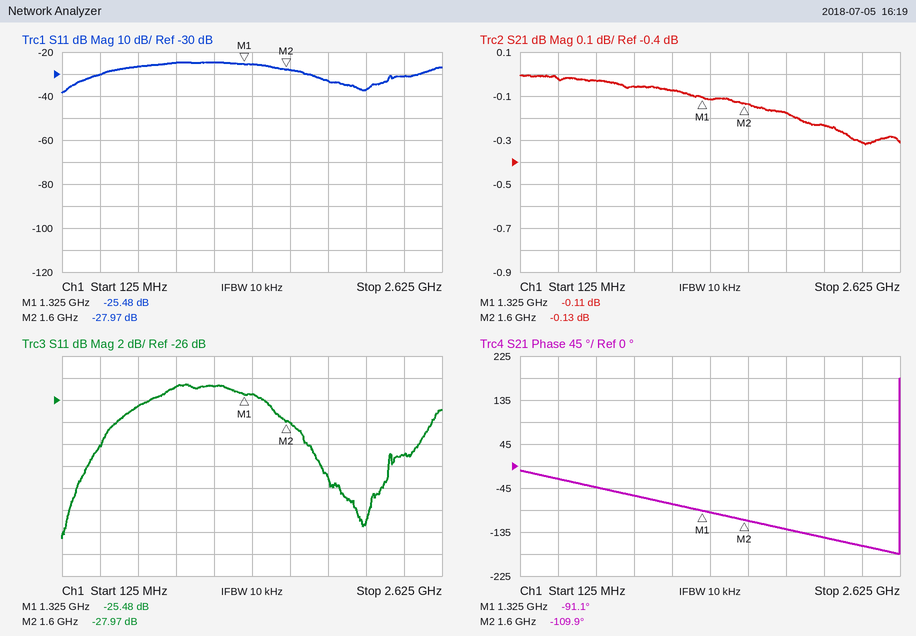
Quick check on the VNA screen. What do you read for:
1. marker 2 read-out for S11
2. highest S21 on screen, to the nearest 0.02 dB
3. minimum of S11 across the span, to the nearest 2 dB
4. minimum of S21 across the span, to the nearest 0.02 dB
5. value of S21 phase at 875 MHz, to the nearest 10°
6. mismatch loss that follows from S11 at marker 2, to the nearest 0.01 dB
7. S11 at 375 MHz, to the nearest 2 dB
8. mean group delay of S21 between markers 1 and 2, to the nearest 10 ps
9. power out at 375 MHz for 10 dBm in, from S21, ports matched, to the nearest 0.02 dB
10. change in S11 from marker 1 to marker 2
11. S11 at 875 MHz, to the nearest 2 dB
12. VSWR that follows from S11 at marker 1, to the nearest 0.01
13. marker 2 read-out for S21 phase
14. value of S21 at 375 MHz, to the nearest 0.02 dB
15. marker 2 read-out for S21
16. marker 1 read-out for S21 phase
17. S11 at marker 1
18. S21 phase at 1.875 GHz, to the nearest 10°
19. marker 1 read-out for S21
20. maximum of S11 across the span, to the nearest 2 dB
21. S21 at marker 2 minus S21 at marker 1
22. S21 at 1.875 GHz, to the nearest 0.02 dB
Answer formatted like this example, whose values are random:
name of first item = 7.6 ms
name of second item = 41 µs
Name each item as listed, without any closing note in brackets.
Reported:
marker 2 read-out for S11 = -27.97 dB
highest S21 on screen, to the nearest 0.02 dB = 0.00 dB
minimum of S11 across the span, to the nearest 2 dB = -38 dB
minimum of S21 across the span, to the nearest 0.02 dB = -0.32 dB
value of S21 phase at 875 MHz, to the nearest 10° = -60°
mismatch loss that follows from S11 at marker 2, to the nearest 0.01 dB = 0.01 dB
S11 at 375 MHz, to the nearest 2 dB = -30 dB
mean group delay of S21 between markers 1 and 2, to the nearest 10 ps = 190 ps
power out at 375 MHz for 10 dBm in, from S21, ports matched, to the nearest 0.02 dB = 9.98 dBm
change in S11 from marker 1 to marker 2 = -2.49 dB
S11 at 875 MHz, to the nearest 2 dB = -24 dB
VSWR that follows from S11 at marker 1, to the nearest 0.01 = 1.11
marker 2 read-out for S21 phase = -109.9°
value of S21 at 375 MHz, to the nearest 0.02 dB = -0.02 dB
marker 2 read-out for S21 = -0.13 dB
marker 1 read-out for S21 phase = -91.1°
S11 at marker 1 = -25.48 dB
S21 phase at 1.875 GHz, to the nearest 10° = -130°
marker 1 read-out for S21 = -0.11 dB
maximum of S11 across the span, to the nearest 2 dB = -24 dB
S21 at marker 2 minus S21 at marker 1 = -0.02 dB
S21 at 1.875 GHz, to the nearest 0.02 dB = -0.18 dB
